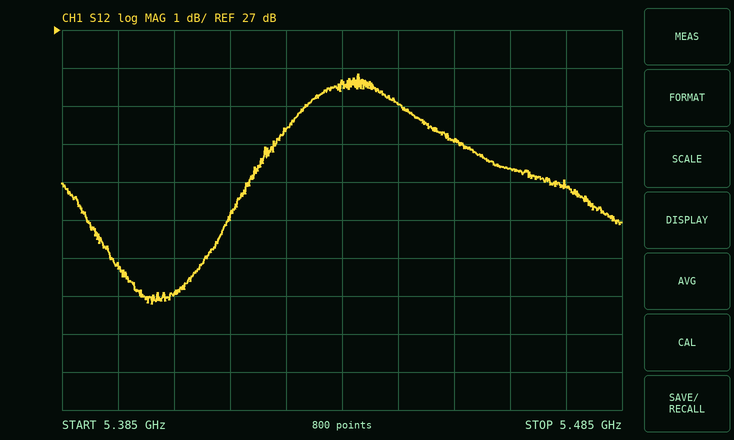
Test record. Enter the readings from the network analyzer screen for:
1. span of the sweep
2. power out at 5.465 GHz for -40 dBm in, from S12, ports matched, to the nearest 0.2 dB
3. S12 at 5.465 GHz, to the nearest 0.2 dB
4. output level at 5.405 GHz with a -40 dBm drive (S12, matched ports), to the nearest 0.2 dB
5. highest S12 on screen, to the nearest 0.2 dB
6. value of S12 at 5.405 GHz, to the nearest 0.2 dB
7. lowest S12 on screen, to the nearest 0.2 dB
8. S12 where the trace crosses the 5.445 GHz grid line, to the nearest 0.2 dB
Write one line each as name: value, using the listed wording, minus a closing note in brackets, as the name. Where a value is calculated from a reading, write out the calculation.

span of the sweep: 100 MHz
power out at 5.465 GHz for -40 dBm in, from S12, ports matched, to the nearest 0.2 dB: -40 dBm + (23.4 dB) = -16.6 dBm
S12 at 5.465 GHz, to the nearest 0.2 dB: 23.4 dB
output level at 5.405 GHz with a -40 dBm drive (S12, matched ports), to the nearest 0.2 dB: -40 dBm + (20.0 dB) = -20.0 dBm
highest S12 on screen, to the nearest 0.2 dB: 25.8 dB
value of S12 at 5.405 GHz, to the nearest 0.2 dB: 20.0 dB
lowest S12 on screen, to the nearest 0.2 dB: 19.8 dB
S12 where the trace crosses the 5.445 GHz grid line, to the nearest 0.2 dB: 25.0 dB
